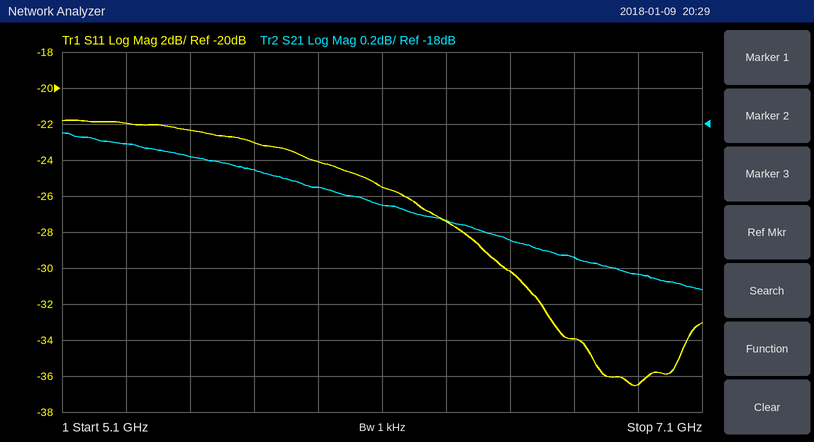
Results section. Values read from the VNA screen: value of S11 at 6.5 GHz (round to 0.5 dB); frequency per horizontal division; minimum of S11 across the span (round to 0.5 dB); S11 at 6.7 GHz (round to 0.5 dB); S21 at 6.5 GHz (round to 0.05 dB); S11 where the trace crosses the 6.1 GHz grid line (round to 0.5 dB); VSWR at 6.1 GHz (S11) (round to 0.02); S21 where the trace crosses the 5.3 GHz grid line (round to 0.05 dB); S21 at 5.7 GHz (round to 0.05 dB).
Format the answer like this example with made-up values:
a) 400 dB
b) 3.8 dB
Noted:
a) -30.0 dB
b) 200 MHz
c) -36.5 dB
d) -34.0 dB
e) -18.65 dB
f) -25.5 dB
g) 1.12
h) -18.10 dB
i) -18.25 dB
